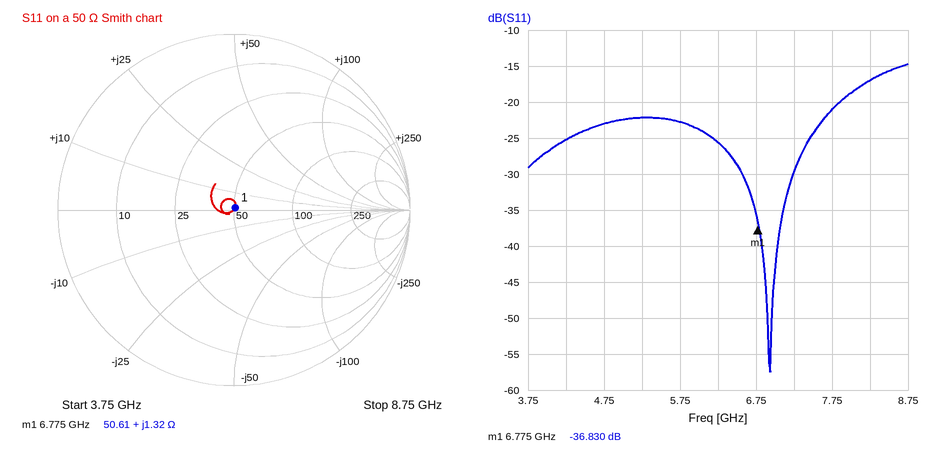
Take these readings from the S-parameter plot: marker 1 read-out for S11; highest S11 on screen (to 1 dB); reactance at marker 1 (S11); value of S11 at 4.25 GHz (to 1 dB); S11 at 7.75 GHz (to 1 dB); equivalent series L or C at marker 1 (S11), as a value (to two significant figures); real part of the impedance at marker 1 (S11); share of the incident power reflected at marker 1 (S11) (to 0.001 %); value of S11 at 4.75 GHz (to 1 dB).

-36.830 dB
-15 dB
+1.32 Ω
-25 dB
-21 dB
31 pH
50.61 Ω
0.021 %
-23 dB
